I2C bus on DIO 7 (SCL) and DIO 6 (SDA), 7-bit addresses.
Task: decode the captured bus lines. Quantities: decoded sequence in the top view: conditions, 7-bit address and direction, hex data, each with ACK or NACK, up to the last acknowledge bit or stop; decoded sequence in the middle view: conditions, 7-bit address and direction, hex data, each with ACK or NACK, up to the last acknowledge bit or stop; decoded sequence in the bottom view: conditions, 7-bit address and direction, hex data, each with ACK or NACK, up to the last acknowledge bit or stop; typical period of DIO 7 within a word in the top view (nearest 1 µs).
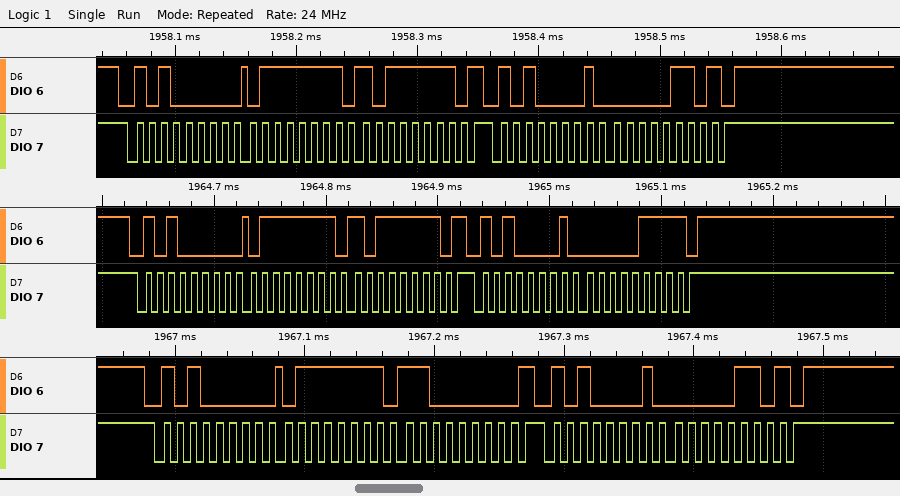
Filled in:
start, address 50 write ACK, 7F ACK, BF ACK, repeated start, address 50 read ACK, 06 NACK, stop
start, address 50 write ACK, 7F ACK, BF ACK, repeated start, address 50 read ACK, 07 NACK, stop
start, address 50 write ACK, 7F ACK, C0 ACK, repeated start, address 50 read ACK, 06 NACK, stop
10 µs
